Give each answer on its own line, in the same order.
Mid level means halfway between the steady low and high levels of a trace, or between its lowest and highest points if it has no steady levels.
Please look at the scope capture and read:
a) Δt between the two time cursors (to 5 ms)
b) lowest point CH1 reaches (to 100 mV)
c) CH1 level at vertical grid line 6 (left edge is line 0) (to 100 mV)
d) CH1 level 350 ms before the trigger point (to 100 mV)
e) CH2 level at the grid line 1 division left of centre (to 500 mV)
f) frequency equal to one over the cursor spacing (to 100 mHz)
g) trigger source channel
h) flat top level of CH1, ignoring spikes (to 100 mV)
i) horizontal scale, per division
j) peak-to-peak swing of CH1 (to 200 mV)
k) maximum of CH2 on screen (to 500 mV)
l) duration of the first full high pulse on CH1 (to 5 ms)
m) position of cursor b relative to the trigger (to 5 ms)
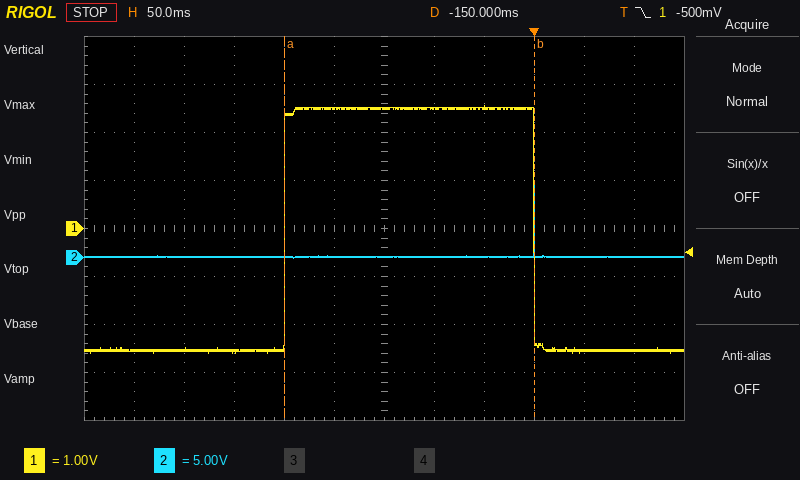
250 ms
-2.6 V
2.5 V
-2.5 V
0.0 V
4.0 Hz
CH1
2.5 V
50 ms
5.2 V
7.5 V
250 ms
0 ms
